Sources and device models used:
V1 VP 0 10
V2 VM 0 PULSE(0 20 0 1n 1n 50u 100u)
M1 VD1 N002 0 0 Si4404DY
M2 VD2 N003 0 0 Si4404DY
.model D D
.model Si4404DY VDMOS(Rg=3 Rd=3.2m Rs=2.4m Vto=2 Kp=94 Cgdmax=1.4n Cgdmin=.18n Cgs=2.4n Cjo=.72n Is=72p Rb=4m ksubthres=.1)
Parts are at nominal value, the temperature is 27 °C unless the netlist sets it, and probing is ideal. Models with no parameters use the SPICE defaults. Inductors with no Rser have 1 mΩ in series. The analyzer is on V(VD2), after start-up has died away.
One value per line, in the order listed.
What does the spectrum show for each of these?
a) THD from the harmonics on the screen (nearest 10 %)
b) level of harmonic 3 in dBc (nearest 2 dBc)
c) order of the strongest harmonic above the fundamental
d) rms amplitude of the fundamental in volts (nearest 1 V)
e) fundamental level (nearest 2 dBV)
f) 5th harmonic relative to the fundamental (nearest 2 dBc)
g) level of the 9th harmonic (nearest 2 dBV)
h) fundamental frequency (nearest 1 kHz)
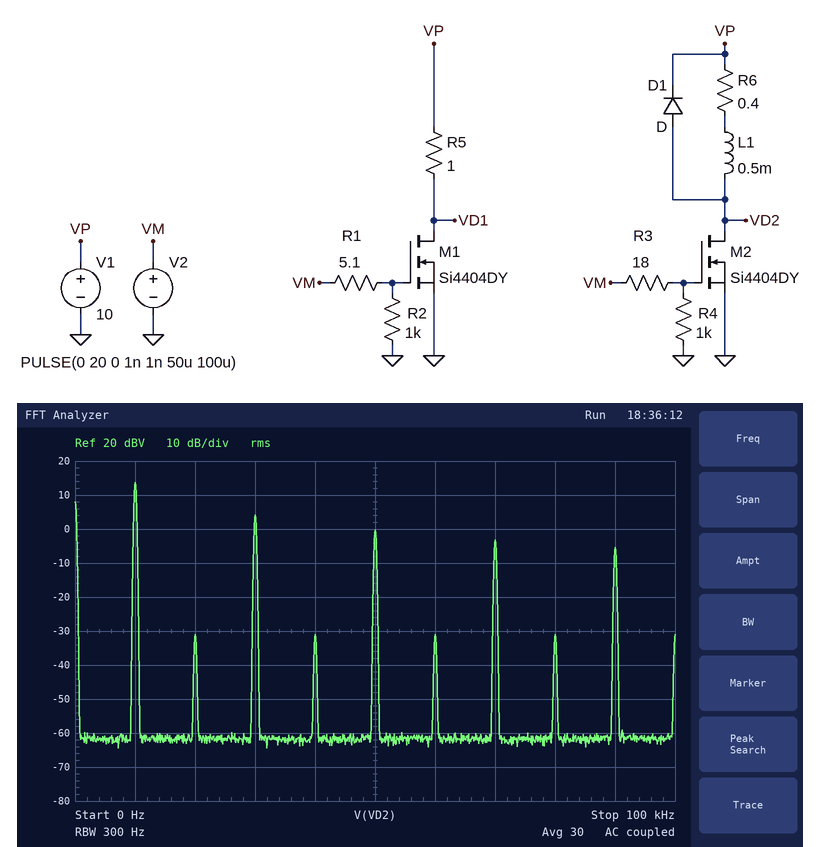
40 %
-10 dBc
3
5 V
14 dBV
-14 dBc
-6 dBV
10 kHz
